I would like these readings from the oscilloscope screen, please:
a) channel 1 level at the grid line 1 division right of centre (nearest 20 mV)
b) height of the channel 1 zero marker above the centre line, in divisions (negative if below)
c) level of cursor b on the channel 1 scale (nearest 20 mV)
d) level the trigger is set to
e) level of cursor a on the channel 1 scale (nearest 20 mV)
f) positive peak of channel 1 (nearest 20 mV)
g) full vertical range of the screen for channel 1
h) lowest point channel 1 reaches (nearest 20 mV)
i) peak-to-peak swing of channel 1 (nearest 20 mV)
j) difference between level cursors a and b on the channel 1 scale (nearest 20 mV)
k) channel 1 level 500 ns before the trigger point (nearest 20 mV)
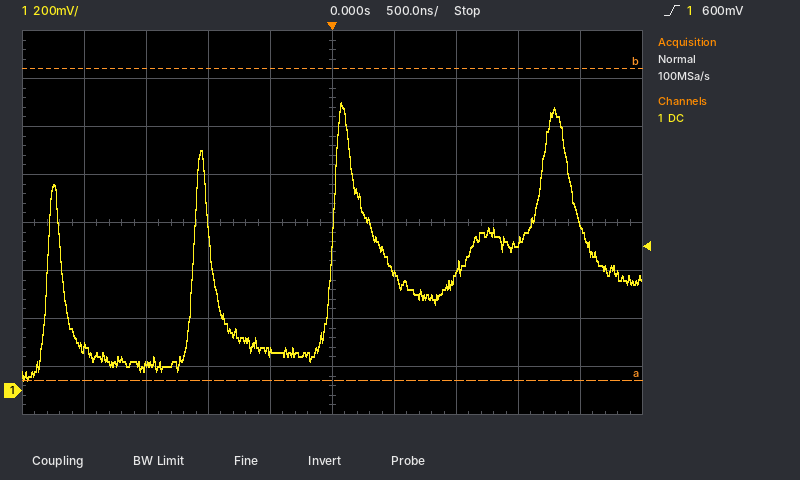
500 mV
-3.5 div
1.34 V
600 mV
40 mV
1.20 V
1.6 V
40 mV
1.16 V
1.30 V
160 mV
